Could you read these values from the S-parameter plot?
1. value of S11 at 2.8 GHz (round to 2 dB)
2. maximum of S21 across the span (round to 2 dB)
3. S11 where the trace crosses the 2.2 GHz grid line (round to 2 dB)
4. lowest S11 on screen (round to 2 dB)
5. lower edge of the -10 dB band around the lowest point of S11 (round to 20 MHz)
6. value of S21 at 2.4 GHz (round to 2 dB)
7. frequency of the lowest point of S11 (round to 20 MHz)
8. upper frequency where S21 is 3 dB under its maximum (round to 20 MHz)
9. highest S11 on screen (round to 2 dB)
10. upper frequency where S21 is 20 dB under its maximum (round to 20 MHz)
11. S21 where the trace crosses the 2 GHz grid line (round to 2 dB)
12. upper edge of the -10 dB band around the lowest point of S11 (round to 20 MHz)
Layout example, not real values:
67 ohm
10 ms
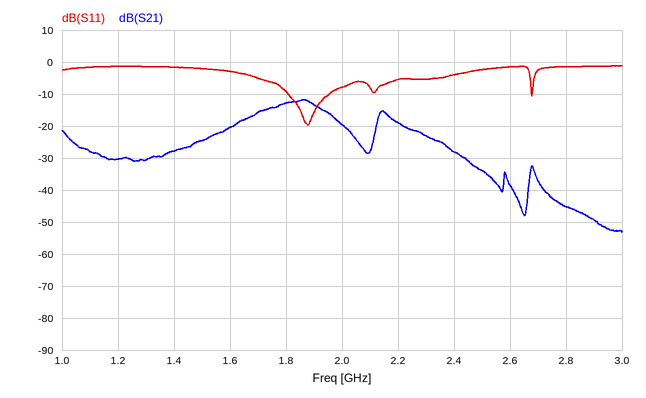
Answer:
-2 dB
-12 dB
-6 dB
-20 dB
1.80 GHz
-28 dB
1.88 GHz
1.92 GHz
-2 dB
2.46 GHz
-20 dB
1.96 GHz
